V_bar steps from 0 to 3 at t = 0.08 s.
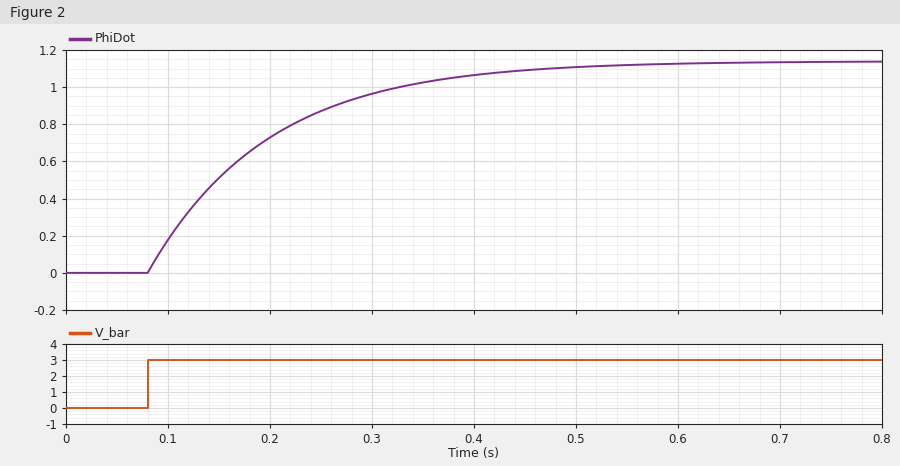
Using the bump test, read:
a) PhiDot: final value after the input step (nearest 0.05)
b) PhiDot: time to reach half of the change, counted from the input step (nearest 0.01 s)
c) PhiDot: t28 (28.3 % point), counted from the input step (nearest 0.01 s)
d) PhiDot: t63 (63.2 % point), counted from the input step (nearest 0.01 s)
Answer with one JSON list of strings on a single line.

["1.15", "0.08 s", "0.04 s", "0.12 s"]
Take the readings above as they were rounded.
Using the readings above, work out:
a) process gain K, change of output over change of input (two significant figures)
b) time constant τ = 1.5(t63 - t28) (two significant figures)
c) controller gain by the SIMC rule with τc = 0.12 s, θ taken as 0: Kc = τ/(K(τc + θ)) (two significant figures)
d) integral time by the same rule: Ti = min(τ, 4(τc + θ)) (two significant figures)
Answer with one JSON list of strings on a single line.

["0.38", "0.12 s", "2.6", "0.12 s"]
